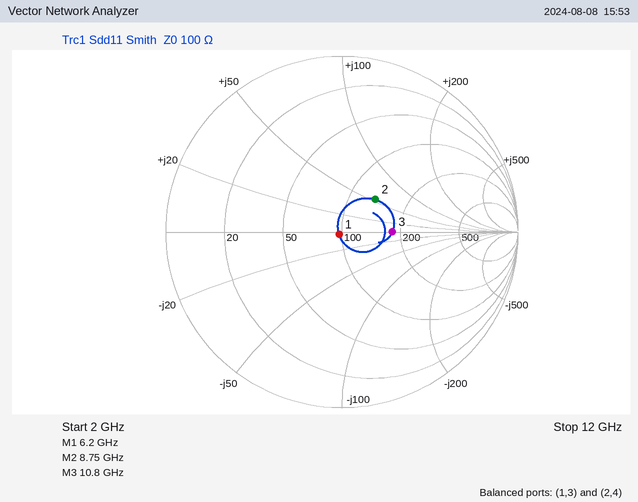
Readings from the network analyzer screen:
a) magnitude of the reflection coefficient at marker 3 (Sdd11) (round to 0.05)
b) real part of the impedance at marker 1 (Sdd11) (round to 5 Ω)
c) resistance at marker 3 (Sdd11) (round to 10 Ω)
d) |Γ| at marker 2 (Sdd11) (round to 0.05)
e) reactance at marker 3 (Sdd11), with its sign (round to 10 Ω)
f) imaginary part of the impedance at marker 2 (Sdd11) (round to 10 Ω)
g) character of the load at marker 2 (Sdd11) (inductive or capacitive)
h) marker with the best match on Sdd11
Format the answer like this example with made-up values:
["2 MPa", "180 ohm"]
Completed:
["0.30", "95 Ω", "180 Ω", "0.25", "0 Ω", "+50 Ω", "inductive", "marker 1"]
